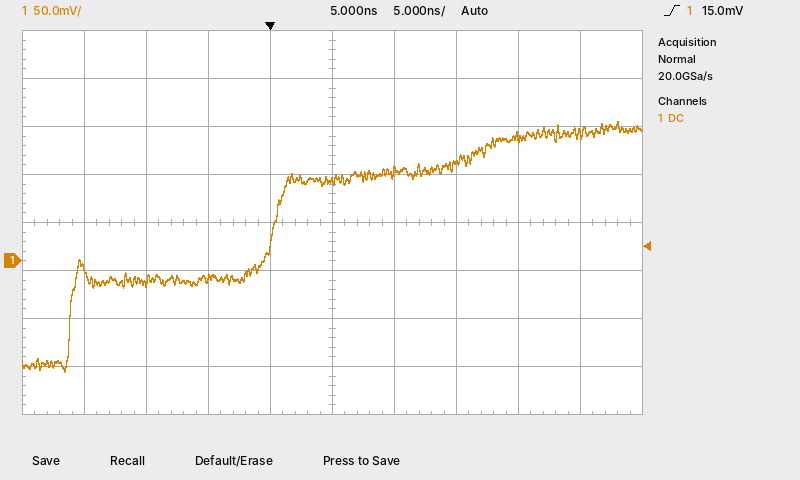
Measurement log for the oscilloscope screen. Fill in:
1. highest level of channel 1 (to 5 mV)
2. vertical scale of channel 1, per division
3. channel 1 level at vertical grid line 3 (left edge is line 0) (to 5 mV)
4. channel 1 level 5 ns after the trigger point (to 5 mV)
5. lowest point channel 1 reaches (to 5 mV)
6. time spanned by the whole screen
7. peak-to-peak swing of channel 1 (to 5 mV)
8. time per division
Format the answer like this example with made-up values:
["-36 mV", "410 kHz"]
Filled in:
["145 mV", "50 mV", "-20 mV", "85 mV", "-115 mV", "50 ns", "260 mV", "5 ns"]
